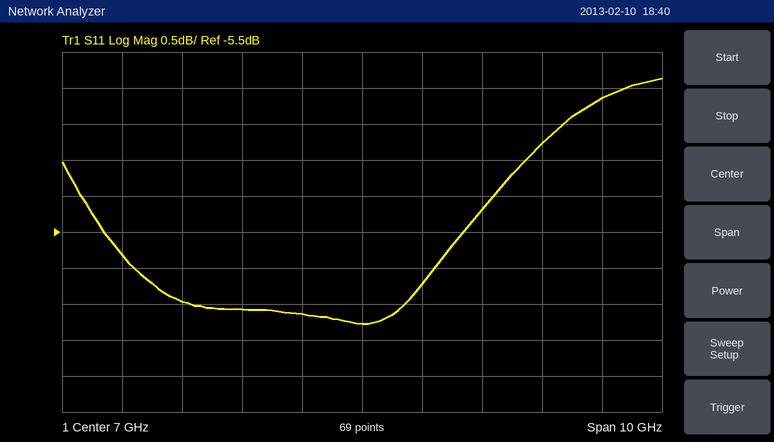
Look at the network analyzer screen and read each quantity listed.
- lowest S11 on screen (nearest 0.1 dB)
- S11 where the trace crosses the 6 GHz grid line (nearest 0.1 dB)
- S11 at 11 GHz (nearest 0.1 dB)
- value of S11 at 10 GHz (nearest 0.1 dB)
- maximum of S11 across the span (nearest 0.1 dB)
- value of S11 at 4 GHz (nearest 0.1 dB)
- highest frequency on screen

-6.8 dB
-6.6 dB
-3.6 dB
-4.3 dB
-3.4 dB
-6.5 dB
12 GHz
